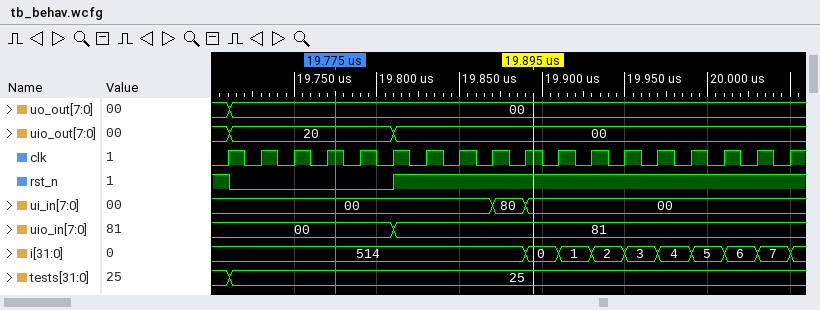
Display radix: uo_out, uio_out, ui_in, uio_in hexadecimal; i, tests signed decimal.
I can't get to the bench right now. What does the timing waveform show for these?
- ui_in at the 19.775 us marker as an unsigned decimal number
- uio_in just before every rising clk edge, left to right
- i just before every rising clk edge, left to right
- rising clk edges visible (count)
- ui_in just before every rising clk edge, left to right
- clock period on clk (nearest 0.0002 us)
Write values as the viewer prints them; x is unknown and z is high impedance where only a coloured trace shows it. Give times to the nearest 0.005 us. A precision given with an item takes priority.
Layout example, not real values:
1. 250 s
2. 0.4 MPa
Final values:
1. 0
2. 00, 00, 00, 00, 00, 00, 81, 81, 81, 81, 81, 81, 81, 81, 81, 81, 81, 81
3. 514, 514, 514, 514, 514, 514, 514, 514, 514, 514, 0, 1, 2, 3, 4, 5, 6, 7
4. 18
5. 00, 00, 00, 00, 00, 00, 00, 00, 00, 80, 00, 00, 00, 00, 00, 00, 00, 00
6. 0.02 us
